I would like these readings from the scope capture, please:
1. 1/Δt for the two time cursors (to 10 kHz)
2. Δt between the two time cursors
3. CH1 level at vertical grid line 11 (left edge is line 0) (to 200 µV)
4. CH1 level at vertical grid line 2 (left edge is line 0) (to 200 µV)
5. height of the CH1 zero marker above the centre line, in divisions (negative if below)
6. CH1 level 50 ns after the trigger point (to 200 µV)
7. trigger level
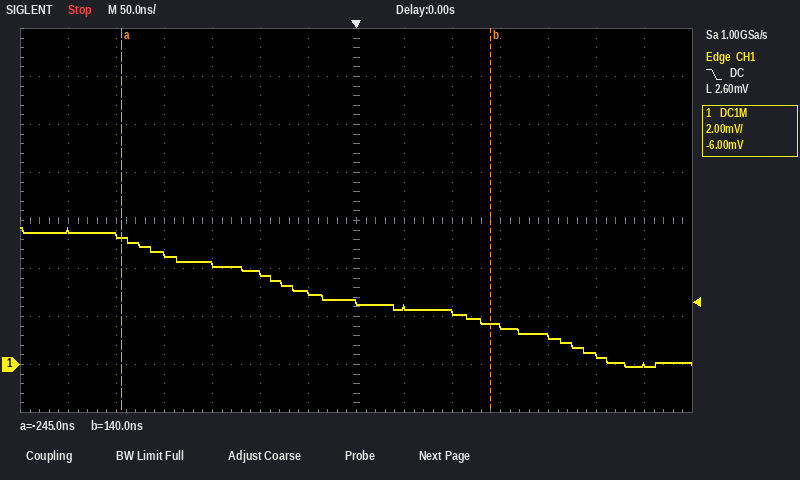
2.60 MHz
385 ns
1.2 mV
5.4 mV
-3.0 div
2.4 mV
2.60 mV
